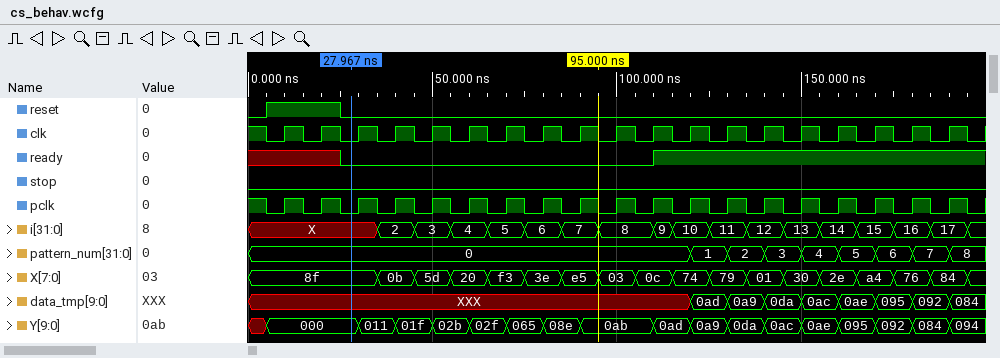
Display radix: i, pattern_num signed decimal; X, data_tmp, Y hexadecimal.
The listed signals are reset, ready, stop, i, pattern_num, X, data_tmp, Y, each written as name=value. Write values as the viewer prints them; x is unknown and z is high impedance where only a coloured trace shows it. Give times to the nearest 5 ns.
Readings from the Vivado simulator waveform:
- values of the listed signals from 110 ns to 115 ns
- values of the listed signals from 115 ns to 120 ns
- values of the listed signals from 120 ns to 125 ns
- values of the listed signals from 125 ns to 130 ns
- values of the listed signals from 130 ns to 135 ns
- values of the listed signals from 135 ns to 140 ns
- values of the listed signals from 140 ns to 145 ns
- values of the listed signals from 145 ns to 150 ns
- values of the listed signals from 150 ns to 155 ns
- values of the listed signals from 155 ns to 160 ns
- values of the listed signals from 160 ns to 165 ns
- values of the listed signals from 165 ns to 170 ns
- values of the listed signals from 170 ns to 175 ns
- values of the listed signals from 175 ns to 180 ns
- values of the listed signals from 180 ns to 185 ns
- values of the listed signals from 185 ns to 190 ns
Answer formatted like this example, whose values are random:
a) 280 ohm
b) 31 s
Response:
a) reset=0, ready=1, stop=0, i=9, pattern_num=0, X=0c, data_tmp=XXX, Y=0ad
b) reset=0, ready=1, stop=0, i=10, pattern_num=0, X=74, data_tmp=XXX, Y=0ad
c) reset=0, ready=1, stop=0, i=10, pattern_num=1, X=74, data_tmp=0ad, Y=0a9
d) reset=0, ready=1, stop=0, i=11, pattern_num=1, X=79, data_tmp=0ad, Y=0a9
e) reset=0, ready=1, stop=0, i=11, pattern_num=2, X=79, data_tmp=0a9, Y=0da
f) reset=0, ready=1, stop=0, i=12, pattern_num=2, X=01, data_tmp=0a9, Y=0da
g) reset=0, ready=1, stop=0, i=12, pattern_num=3, X=01, data_tmp=0da, Y=0ac
h) reset=0, ready=1, stop=0, i=13, pattern_num=3, X=30, data_tmp=0da, Y=0ac
i) reset=0, ready=1, stop=0, i=13, pattern_num=4, X=30, data_tmp=0ac, Y=0ae
j) reset=0, ready=1, stop=0, i=14, pattern_num=4, X=2e, data_tmp=0ac, Y=0ae
k) reset=0, ready=1, stop=0, i=14, pattern_num=5, X=2e, data_tmp=0ae, Y=095
l) reset=0, ready=1, stop=0, i=15, pattern_num=5, X=a4, data_tmp=0ae, Y=095
m) reset=0, ready=1, stop=0, i=15, pattern_num=6, X=a4, data_tmp=095, Y=092
n) reset=0, ready=1, stop=0, i=16, pattern_num=6, X=76, data_tmp=095, Y=092
o) reset=0, ready=1, stop=0, i=16, pattern_num=7, X=76, data_tmp=092, Y=084
p) reset=0, ready=1, stop=0, i=17, pattern_num=7, X=84, data_tmp=092, Y=084
